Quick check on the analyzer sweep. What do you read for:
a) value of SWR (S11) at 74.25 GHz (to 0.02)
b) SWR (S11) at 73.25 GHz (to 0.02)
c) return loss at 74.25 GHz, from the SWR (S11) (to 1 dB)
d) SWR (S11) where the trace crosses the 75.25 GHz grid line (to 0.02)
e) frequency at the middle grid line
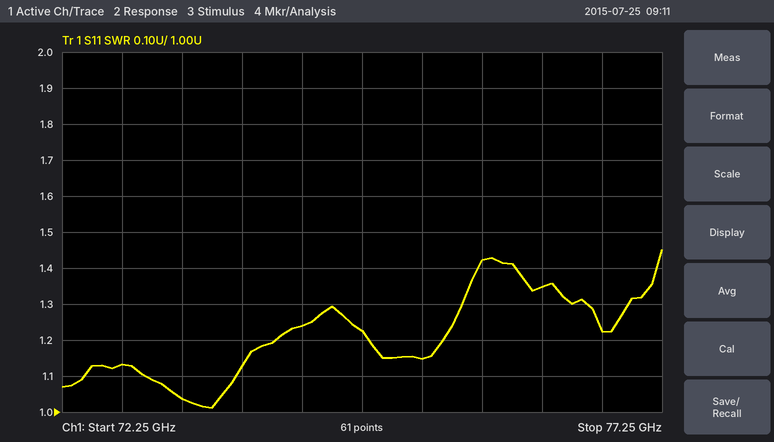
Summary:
1.24
1.04
19 dB
1.14
74.75 GHz
